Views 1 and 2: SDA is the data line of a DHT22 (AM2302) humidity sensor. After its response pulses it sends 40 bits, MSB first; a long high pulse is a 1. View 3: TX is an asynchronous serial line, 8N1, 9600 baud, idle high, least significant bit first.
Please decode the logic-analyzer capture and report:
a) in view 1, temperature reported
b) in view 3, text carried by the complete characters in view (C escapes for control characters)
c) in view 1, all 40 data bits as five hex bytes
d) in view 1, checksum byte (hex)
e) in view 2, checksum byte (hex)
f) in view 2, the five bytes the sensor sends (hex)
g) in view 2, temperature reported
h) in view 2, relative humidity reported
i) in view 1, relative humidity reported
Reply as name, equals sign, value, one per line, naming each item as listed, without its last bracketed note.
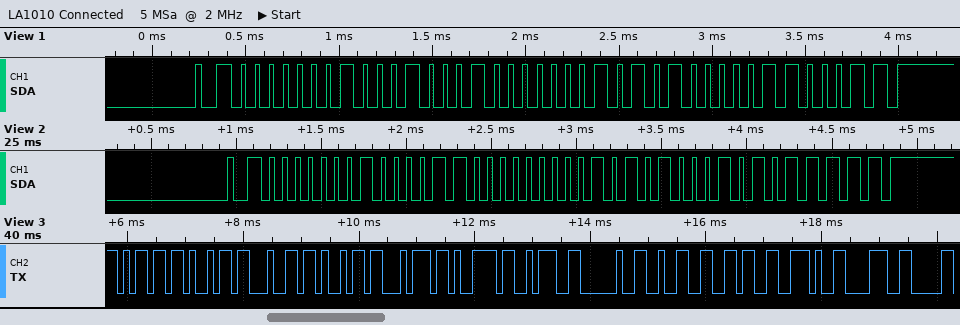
in view 1, temperature reported = 33.6 °C
in view 3, text carried by the complete characters in view = "midity: 26.8"
in view 1, all 40 data bits as five hex bytes = 01 11 01 50 63
in view 1, checksum byte = 0x63
in view 2, checksum byte = 0x5F
in view 2, the five bytes the sensor sends = 01 0C 01 51 5F
in view 2, temperature reported = 33.7 °C
in view 2, relative humidity reported = 26.8 %
in view 1, relative humidity reported = 27.3 %
